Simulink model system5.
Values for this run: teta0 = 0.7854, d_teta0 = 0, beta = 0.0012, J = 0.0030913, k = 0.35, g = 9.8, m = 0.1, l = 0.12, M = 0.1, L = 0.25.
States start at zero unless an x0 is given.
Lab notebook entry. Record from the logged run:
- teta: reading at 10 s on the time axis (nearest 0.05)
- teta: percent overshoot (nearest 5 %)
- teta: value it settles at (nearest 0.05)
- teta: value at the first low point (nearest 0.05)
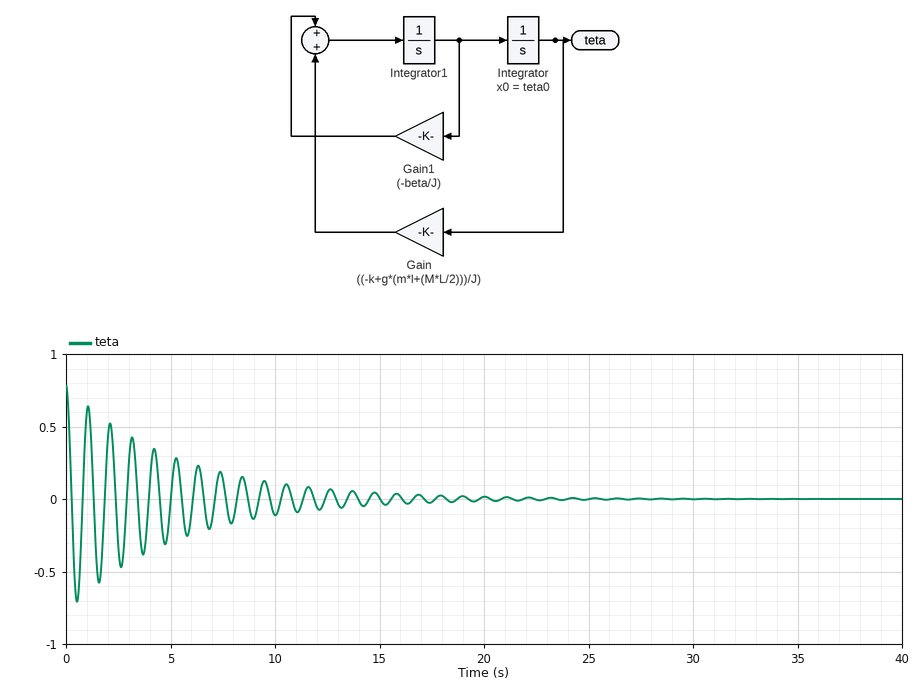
-0.10
90 %
0.00
-0.70
